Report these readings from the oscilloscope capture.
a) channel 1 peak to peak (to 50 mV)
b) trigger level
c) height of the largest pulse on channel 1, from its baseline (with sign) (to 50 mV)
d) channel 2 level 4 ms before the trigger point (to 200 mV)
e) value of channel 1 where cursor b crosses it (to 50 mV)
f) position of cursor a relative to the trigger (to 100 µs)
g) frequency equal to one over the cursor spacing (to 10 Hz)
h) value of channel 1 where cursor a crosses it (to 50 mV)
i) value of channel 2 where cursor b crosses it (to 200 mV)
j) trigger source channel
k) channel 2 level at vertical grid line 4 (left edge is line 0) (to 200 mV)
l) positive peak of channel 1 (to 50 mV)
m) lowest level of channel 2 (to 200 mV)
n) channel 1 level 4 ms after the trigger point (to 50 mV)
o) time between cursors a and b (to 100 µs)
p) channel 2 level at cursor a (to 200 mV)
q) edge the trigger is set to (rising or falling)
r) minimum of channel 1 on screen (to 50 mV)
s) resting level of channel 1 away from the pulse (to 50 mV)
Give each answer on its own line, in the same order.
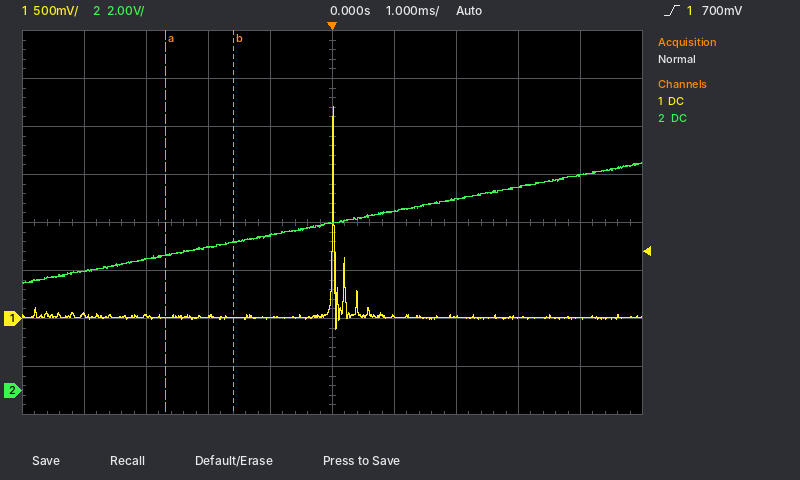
2.30 V
700 mV
+2.20 V
5.0 V
0 mV
-2.7 ms
910 Hz
0 mV
6.2 V
channel 1
6.4 V
2.20 V
4.4 V
0 mV
1.1 ms
5.6 V
rising
-100 mV
0 mV
